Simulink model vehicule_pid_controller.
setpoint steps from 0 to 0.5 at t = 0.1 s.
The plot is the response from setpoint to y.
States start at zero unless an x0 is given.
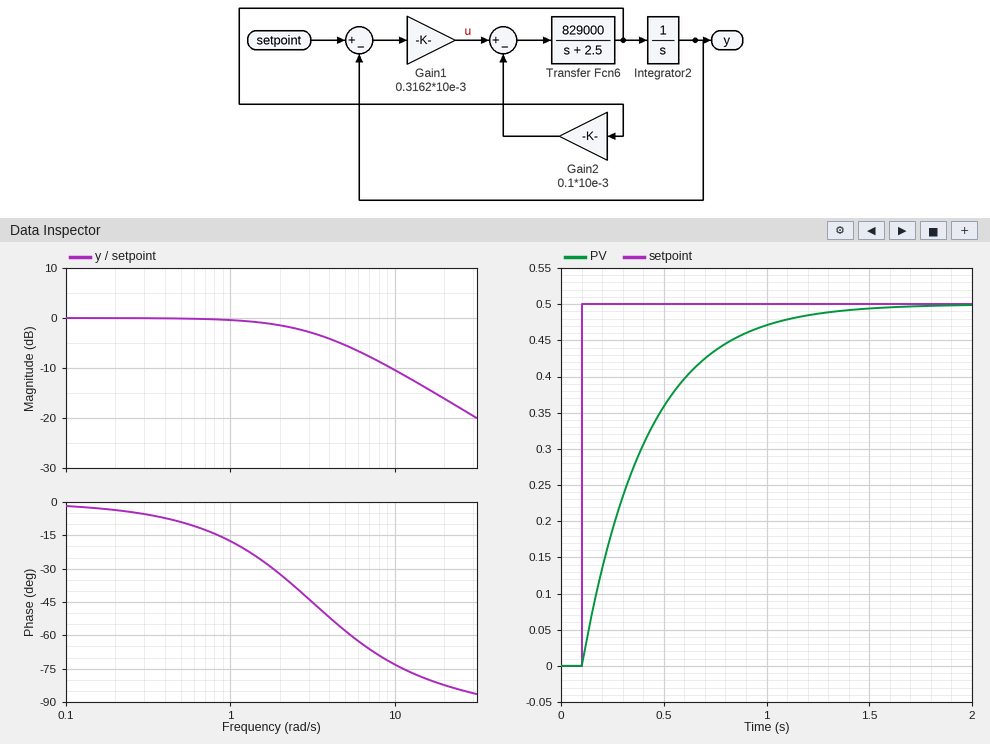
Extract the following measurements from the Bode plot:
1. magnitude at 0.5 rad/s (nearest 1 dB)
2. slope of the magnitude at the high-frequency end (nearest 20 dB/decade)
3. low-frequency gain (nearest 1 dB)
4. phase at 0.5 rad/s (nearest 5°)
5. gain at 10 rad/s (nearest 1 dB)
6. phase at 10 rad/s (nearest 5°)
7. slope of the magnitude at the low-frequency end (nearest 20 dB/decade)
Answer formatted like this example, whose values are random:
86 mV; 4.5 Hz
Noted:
0 dB; -20 dB/decade; 0 dB; -10°; -10 dB; -75°; 0 dB/decade
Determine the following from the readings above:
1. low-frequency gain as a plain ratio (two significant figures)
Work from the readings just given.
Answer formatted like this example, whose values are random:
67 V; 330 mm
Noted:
1.0
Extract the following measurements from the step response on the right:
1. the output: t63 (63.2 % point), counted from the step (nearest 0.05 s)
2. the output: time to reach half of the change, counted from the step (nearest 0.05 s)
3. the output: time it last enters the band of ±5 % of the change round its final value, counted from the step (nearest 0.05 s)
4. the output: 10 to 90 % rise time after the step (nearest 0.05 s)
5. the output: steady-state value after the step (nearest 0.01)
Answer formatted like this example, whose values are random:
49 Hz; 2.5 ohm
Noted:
0.30 s; 0.20 s; 0.95 s; 0.70 s; 0.50
